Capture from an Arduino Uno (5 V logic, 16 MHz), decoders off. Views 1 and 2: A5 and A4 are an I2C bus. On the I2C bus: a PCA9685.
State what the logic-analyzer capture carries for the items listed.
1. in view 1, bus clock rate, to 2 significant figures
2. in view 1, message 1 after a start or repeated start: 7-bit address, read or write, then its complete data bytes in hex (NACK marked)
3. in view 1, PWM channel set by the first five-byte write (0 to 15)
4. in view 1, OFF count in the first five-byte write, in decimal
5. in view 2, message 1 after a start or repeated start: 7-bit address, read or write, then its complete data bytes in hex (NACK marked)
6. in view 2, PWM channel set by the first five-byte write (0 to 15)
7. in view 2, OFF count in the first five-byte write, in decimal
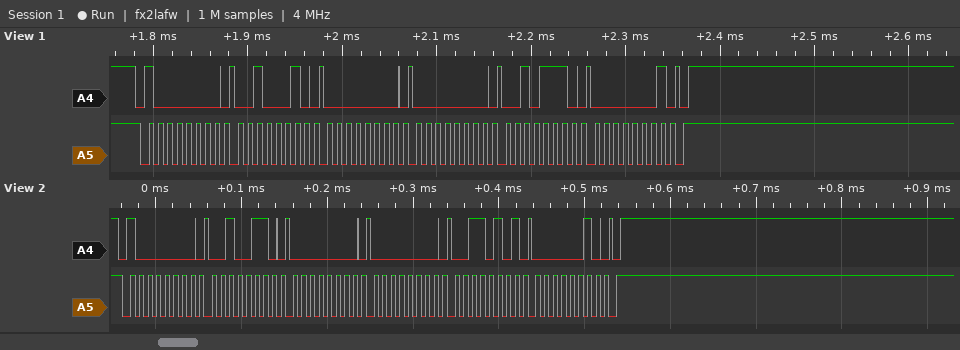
100 kHz
0x40 write: 22 00 00 2E 01
7
302
0x40 write: 26 00 00 35 02
8
565
